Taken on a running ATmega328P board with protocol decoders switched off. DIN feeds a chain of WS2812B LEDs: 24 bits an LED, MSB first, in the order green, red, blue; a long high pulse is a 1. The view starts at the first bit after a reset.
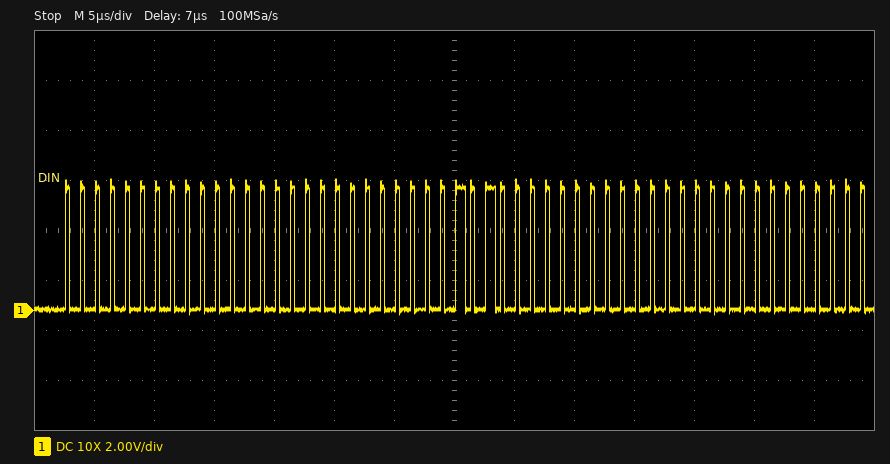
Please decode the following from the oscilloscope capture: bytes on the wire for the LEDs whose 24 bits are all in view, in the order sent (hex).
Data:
00 00 00 28 00 00
